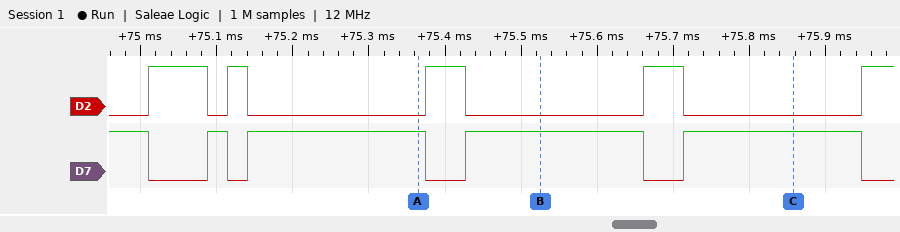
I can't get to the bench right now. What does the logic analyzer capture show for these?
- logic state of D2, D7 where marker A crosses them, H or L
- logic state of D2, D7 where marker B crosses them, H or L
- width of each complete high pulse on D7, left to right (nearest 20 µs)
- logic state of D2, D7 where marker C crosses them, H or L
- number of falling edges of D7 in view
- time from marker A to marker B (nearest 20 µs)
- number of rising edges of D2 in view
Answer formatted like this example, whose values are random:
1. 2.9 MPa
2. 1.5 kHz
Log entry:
1. D2=L, D7=H
2. D2=L, D7=H
3. 20 µs, 240 µs, 240 µs, 240 µs
4. D2=L, D7=H
5. 5
6. 160 µs
7. 5
